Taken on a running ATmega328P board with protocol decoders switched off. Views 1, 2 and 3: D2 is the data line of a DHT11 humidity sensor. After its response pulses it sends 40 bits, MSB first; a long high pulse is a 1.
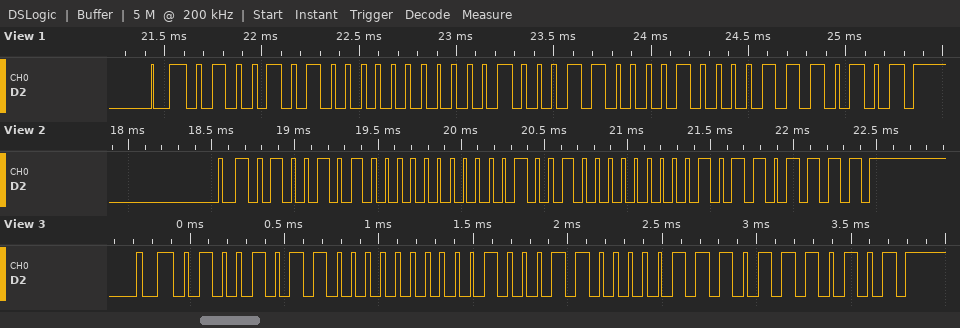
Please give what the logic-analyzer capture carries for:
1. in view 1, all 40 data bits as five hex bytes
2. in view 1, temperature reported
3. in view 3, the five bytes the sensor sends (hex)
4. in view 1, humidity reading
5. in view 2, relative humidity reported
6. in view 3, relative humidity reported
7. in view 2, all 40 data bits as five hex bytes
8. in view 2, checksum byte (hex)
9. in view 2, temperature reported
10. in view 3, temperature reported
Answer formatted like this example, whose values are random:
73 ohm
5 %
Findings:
4A 00 23 08 75
35.8 °C
4B 00 23 07 75
74 %
74 %
75 %
4A 00 24 01 6F
0x6F
36.1 °C
35.7 °C
